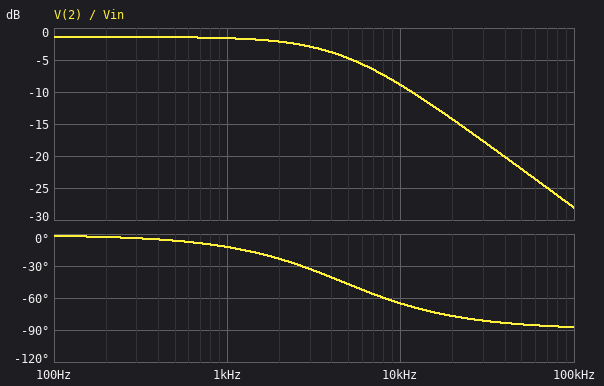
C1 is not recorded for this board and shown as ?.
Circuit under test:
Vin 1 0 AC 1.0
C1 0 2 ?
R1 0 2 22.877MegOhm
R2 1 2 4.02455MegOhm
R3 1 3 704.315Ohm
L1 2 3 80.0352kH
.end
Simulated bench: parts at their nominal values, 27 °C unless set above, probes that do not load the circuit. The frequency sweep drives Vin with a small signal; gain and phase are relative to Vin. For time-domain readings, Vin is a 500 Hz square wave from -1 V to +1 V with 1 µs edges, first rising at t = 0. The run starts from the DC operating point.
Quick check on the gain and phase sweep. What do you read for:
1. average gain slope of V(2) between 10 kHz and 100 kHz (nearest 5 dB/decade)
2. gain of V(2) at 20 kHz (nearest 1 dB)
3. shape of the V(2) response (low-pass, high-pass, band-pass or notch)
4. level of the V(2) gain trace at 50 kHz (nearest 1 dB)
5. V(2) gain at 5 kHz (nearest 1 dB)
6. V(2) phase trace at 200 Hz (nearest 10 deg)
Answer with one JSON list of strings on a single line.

["-20 dB/decade", "-14 dB", "low-pass", "-22 dB", "-5 dB", "0 deg"]
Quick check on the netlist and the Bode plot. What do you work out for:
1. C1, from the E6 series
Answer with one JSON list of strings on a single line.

["10 pF"]
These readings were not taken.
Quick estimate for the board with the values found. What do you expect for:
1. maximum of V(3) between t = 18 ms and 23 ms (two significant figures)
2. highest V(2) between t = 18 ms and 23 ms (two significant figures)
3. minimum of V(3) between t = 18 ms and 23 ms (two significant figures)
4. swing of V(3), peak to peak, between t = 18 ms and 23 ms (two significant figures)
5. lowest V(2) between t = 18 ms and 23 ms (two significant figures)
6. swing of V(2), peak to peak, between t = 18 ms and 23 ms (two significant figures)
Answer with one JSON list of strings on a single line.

["1.0 V", "800 mV", "-1.0 V", "2.0 V", "-920 mV", "1.7 V"]
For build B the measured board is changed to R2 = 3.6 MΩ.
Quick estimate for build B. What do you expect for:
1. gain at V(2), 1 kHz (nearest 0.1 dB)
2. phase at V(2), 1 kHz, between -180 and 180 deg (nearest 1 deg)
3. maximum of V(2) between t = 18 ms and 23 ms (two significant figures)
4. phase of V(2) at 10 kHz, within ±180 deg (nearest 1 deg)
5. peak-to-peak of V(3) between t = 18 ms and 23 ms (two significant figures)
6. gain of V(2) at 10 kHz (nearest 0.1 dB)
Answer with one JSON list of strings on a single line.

["-1.4 dB", "-11 deg", "810 mV", "-63 deg", "2.0 V", "-8.1 dB"]
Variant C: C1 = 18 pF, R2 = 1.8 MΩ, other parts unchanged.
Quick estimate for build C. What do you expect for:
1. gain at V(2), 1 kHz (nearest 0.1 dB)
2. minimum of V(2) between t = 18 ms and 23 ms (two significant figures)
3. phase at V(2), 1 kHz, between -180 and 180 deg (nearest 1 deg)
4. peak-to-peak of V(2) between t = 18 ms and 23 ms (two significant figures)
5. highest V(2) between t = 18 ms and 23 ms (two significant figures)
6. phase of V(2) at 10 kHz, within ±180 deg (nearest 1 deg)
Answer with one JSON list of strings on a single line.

["-0.8 dB", "-980 mV", "-11 deg", "1.9 V", "880 mV", "-62 deg"]
